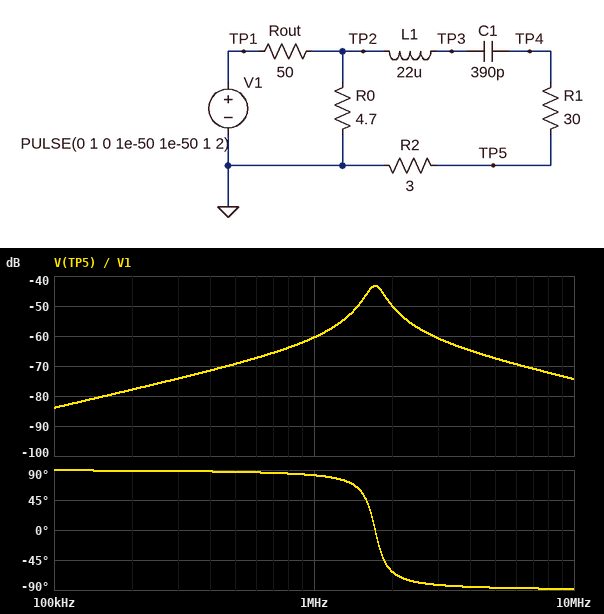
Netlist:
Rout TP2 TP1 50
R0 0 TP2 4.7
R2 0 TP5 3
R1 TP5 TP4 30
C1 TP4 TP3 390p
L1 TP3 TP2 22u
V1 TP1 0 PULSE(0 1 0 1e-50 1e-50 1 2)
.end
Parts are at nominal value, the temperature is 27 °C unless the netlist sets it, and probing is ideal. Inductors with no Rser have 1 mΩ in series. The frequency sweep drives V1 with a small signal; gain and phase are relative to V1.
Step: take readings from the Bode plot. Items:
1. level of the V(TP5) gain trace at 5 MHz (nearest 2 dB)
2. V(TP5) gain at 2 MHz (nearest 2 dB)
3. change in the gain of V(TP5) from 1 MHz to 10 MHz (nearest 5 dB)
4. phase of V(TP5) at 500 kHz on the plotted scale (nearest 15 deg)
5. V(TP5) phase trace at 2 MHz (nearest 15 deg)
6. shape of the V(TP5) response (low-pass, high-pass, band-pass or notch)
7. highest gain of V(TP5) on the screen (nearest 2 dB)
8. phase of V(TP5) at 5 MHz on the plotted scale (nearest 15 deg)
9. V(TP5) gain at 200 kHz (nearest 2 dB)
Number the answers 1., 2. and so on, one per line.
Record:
1. -68 dB
2. -50 dB
3. -15 dB
4. 90 deg
5. -60 deg
6. band-pass
7. -44 dB
8. -90 deg
9. -78 dB
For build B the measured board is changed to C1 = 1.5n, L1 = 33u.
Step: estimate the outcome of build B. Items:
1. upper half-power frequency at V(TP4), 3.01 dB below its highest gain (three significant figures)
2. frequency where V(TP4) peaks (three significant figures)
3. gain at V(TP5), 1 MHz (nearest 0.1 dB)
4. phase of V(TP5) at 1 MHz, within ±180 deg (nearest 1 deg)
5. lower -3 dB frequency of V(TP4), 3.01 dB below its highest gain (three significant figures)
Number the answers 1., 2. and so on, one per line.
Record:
1. 811 kHz
2. 715 kHz
3. -52.4 dB
4. -70 deg
5. 631 kHz
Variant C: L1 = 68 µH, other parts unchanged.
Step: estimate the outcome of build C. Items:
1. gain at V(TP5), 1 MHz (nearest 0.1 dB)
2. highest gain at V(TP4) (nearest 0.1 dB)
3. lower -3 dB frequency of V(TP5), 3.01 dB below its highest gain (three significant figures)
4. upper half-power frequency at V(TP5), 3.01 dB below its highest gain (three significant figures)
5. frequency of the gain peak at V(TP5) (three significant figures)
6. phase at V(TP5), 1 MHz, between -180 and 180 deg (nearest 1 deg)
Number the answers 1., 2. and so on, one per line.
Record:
1. -44.2 dB
2. -22.4 dB
3. 935 kHz
4. 1.02 MHz
5. 977 kHz
6. -27 deg
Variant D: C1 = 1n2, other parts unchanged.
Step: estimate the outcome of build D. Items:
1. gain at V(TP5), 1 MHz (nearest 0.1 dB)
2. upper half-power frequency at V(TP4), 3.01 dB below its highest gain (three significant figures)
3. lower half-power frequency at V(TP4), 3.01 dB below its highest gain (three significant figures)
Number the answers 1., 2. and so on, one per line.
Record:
1. -43.3 dB
2. 1.12 MHz
3. 854 kHz
